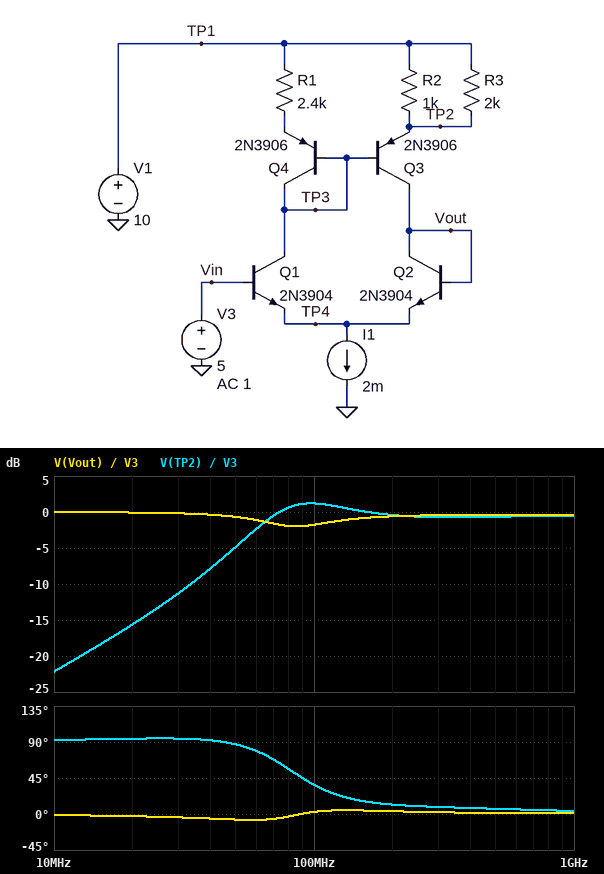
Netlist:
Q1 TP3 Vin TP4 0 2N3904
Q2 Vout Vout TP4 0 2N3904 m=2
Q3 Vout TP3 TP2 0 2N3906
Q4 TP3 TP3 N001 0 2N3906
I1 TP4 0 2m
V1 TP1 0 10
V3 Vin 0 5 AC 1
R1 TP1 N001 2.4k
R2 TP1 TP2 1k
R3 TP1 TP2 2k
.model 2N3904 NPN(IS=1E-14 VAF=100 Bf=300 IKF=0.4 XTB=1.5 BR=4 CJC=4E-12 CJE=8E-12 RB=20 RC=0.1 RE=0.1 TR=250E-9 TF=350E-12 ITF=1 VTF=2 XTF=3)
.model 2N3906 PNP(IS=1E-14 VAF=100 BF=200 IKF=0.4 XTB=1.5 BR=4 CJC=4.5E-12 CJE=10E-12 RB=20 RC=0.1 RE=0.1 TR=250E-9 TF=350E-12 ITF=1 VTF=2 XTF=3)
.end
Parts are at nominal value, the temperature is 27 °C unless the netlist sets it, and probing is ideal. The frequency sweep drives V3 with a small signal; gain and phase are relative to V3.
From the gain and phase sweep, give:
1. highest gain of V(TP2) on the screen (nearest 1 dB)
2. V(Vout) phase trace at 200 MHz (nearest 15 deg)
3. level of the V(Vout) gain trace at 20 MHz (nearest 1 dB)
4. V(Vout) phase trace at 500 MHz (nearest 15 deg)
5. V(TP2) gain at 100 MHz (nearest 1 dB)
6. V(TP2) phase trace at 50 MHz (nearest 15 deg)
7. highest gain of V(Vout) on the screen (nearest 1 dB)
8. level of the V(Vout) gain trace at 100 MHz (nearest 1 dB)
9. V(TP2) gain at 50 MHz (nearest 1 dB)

1 dB
0 deg
0 dB
0 deg
1 dB
90 deg
0 dB
-2 dB
-5 dB
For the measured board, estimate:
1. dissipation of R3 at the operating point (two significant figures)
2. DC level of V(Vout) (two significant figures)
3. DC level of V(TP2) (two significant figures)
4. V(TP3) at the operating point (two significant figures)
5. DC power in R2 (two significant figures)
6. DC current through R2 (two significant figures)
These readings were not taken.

540 µW
5.0 V
9.0 V
8.3 V
1.1 mW
1.0 mA
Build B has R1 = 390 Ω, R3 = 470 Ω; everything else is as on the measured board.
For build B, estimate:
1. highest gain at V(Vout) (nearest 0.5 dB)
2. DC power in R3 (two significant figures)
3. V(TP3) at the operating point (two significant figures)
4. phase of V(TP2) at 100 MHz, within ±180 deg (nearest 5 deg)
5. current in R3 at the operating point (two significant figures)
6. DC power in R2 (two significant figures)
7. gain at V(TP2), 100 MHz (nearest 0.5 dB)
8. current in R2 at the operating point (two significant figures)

0 dB
260 µW
9.0 V
90 deg
740 µA
120 µW
-7.5 dB
350 µA
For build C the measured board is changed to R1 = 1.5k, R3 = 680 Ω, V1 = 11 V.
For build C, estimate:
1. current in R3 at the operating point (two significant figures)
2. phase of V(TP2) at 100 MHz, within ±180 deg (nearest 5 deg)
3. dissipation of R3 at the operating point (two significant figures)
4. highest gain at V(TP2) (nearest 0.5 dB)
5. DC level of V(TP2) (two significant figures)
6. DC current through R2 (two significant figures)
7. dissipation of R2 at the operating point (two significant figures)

930 µA
65 deg
580 µW
0.5 dB
10 V
630 µA
400 µW
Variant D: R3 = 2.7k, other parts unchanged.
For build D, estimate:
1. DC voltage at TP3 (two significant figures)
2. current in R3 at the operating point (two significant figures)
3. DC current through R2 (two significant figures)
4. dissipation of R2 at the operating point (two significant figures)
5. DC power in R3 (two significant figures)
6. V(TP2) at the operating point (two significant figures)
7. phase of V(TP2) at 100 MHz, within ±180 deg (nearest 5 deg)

8.2 V
410 µA
1.1 mA
1.2 mW
460 µW
8.9 V
35 deg
